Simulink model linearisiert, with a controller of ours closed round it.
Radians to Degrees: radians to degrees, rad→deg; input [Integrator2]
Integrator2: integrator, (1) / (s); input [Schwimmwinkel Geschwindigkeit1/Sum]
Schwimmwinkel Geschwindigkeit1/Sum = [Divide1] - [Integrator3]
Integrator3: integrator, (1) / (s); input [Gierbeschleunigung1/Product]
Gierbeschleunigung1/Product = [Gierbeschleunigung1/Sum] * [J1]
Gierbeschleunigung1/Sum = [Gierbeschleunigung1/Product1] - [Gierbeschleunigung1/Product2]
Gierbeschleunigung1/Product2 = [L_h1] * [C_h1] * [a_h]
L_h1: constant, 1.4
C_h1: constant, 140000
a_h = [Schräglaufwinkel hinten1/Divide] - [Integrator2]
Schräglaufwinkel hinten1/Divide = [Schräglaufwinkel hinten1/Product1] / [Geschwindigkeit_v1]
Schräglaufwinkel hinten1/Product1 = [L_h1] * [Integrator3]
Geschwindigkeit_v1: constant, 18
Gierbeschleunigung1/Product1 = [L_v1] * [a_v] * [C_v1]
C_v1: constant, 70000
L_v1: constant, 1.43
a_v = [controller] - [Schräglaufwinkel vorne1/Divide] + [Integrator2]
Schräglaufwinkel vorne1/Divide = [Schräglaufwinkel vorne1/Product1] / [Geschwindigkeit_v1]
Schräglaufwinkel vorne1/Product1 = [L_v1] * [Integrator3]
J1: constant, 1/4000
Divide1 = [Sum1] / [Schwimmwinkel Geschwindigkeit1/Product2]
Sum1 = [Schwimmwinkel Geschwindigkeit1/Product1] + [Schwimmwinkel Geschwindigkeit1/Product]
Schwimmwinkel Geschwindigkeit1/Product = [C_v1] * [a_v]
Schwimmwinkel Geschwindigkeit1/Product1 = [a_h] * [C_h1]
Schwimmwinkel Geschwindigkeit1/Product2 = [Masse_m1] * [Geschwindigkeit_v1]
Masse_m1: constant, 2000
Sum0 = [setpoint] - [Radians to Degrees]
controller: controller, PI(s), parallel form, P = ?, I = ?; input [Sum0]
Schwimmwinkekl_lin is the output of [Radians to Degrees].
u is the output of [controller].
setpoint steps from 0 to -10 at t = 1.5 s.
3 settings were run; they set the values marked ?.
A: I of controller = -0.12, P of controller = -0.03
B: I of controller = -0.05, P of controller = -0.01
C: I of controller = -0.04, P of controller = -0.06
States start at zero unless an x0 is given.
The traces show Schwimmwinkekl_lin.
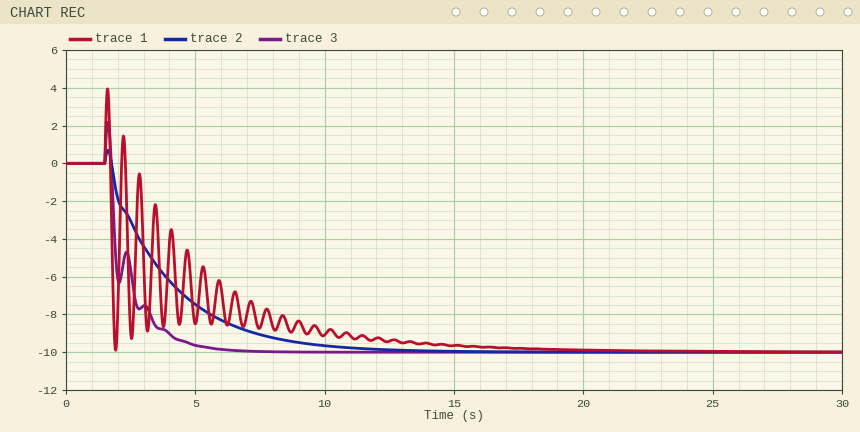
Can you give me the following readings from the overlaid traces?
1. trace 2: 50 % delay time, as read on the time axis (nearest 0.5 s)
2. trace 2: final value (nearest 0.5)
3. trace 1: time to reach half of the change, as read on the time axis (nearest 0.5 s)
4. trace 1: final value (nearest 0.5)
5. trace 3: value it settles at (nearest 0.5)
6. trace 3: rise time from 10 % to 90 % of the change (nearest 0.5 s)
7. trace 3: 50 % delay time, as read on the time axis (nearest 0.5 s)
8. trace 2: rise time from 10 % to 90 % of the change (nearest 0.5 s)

3.5 s
-10.0
2.0 s
-10.0
-10.0
2.0 s
2.0 s
5.5 s
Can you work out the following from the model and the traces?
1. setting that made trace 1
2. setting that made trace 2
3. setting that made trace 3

C
B
A
